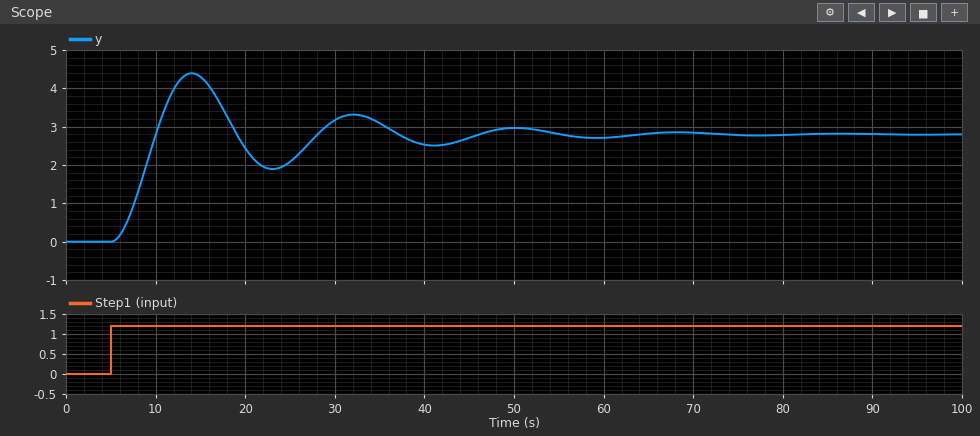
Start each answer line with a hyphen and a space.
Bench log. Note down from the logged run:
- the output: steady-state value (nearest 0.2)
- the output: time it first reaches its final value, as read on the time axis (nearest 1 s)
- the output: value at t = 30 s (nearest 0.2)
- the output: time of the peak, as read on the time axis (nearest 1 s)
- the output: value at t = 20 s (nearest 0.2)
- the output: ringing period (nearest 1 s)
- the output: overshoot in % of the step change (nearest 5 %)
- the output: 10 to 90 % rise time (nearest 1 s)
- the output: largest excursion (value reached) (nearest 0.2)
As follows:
- 2.8
- 10 s
- 3.2
- 14 s
- 2.4
- 18 s
- 55 %
- 3 s
- 4.4
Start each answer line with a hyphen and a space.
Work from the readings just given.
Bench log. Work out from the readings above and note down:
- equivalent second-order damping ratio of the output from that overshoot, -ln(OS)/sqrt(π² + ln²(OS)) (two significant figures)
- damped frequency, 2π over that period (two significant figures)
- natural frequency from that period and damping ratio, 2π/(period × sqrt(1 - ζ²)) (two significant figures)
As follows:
- 0.19
- 0.35 rad/s
- 0.36 rad/s
